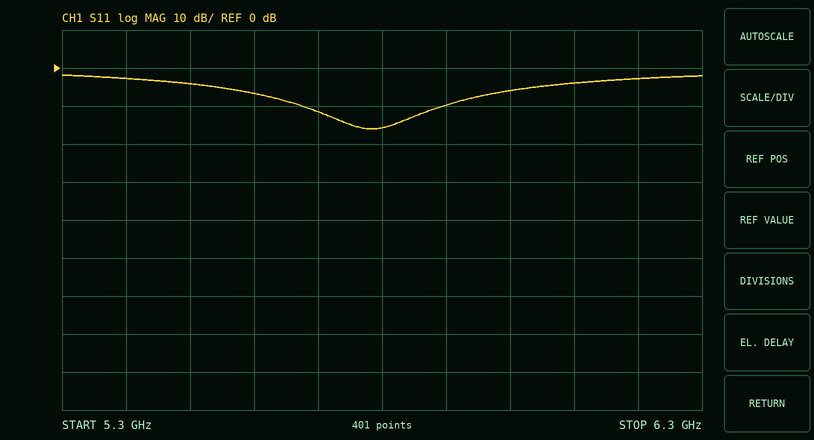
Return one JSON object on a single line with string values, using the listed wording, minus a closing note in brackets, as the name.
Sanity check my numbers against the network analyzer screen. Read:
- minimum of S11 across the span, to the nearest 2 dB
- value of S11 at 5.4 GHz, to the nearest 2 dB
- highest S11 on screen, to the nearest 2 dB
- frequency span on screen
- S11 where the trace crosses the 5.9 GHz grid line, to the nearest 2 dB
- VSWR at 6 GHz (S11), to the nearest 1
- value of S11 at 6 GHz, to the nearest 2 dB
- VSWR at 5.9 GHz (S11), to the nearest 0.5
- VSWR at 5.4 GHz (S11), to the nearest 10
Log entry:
{"minimum of S11 across the span, to the nearest 2 dB": "-16 dB", "value of S11 at 5.4 GHz, to the nearest 2 dB": "-2 dB", "highest S11 on screen, to the nearest 2 dB": "-2 dB", "frequency span on screen": "1 GHz", "S11 where the trace crosses the 5.9 GHz grid line, to the nearest 2 dB": "-10 dB", "VSWR at 6 GHz (S11), to the nearest 1": "3", "value of S11 at 6 GHz, to the nearest 2 dB": "-6 dB", "VSWR at 5.9 GHz (S11), to the nearest 0.5": "2.0", "VSWR at 5.4 GHz (S11), to the nearest 10": "10"}
